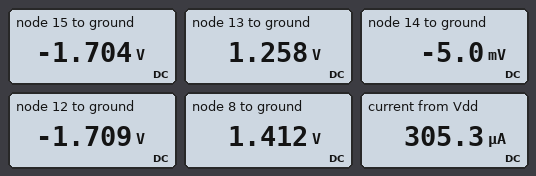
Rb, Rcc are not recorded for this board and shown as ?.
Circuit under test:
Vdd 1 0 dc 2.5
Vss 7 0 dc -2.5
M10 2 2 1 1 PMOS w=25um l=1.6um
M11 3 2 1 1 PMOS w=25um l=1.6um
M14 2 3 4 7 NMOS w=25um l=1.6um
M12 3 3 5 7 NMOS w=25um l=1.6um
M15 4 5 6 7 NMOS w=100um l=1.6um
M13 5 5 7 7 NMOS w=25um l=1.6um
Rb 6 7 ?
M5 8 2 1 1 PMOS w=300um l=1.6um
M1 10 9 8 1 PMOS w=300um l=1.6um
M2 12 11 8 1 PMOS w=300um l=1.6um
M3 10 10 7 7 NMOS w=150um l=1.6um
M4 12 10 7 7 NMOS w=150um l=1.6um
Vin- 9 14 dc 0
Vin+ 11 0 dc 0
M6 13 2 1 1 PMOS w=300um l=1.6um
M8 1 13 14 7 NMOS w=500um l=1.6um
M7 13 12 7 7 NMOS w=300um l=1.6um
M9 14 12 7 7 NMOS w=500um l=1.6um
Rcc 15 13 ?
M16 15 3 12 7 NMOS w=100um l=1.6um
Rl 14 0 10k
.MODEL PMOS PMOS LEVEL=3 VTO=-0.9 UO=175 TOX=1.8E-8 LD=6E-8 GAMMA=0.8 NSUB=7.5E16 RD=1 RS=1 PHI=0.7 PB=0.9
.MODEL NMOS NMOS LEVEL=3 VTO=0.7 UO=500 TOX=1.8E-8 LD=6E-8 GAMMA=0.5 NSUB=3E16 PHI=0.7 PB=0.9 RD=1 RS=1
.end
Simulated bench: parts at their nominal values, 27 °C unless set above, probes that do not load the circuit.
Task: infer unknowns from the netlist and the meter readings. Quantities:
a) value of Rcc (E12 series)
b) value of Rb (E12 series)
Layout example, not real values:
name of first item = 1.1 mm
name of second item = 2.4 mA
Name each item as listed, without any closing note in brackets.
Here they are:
value of Rcc = 820 kΩ
value of Rb = 5.6 kΩ
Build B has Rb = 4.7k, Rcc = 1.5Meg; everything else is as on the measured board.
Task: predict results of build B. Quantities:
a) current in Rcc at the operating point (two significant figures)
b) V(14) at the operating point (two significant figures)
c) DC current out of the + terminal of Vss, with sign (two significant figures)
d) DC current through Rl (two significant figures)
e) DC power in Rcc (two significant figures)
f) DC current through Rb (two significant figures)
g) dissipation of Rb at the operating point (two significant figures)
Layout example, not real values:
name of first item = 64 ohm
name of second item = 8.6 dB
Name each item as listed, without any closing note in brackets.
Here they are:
current in Rcc at the operating point = 2.0 µA
V(14) at the operating point = -2.3 mV
DC current out of the + terminal of Vss, with sign = -440 µA
DC current through Rl = 230 nA
DC power in Rcc = 5.9 µW
DC current through Rb = 9.7 µA
dissipation of Rb at the operating point = 440 nW
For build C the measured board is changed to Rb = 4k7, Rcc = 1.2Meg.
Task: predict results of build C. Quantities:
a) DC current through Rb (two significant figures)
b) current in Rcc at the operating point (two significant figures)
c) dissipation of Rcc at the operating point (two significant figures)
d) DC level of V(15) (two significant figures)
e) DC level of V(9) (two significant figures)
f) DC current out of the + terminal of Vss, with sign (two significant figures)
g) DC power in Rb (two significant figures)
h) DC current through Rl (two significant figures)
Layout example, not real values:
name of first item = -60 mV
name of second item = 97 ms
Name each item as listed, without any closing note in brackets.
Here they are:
DC current through Rb = 9.7 µA
current in Rcc at the operating point = 2.5 µA
dissipation of Rcc at the operating point = 7.3 µW
DC level of V(15) = -1.7 V
DC level of V(9) = -2.9 mV
DC current out of the + terminal of Vss, with sign = -440 µA
DC power in Rb = 440 nW
DC current through Rl = 290 nA
